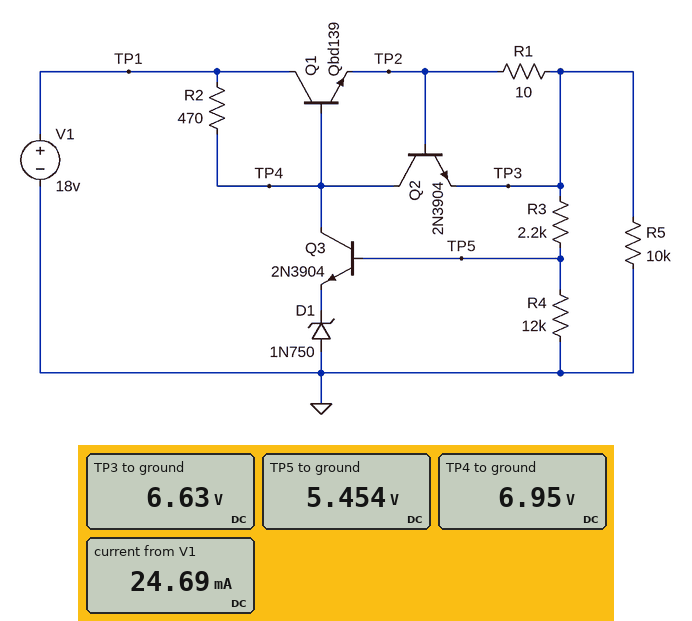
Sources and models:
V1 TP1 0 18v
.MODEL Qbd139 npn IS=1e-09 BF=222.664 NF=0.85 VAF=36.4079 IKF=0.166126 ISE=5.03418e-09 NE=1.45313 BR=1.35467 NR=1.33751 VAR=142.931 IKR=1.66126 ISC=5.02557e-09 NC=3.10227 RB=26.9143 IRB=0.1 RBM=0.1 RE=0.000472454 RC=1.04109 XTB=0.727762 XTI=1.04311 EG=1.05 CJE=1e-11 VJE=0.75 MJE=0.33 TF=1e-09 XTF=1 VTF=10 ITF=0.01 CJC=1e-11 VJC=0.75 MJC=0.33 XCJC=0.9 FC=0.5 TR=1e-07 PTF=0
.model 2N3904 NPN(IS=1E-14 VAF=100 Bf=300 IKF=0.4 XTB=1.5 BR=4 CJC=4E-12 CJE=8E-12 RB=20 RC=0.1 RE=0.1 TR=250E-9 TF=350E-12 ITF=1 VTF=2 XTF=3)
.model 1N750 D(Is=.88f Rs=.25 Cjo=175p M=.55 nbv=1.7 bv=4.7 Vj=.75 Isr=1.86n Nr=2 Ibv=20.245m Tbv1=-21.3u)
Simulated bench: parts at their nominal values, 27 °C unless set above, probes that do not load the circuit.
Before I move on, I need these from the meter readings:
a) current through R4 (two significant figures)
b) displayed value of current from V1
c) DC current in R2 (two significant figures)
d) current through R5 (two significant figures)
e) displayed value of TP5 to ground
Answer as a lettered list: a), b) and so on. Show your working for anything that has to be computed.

a) (5.454 V) / 12 kΩ = 450 µA
b) 24.69 mA
c) (18 V - 6.95 V) / 470 Ω = 24 mA
d) (6.63 V) / 10 kΩ = 660 µA
e) 5.454 V
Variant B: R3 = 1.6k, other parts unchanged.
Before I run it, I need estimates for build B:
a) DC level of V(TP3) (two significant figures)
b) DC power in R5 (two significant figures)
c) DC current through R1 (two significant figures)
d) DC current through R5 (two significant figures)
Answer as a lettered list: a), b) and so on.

a) 6.3 V
b) 4.0 mW
c) 1.2 mA
d) 630 µA
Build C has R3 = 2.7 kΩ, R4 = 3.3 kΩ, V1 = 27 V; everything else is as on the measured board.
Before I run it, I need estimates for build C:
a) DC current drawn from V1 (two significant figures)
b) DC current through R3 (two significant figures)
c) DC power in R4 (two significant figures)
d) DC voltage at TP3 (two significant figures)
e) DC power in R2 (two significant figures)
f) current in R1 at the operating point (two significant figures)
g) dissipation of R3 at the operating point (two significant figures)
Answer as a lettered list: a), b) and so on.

a) 38 mA
b) 1.8 mA
c) 9.1 mW
d) 10 V
e) 570 mW
f) 2.8 mA
g) 8.6 mW
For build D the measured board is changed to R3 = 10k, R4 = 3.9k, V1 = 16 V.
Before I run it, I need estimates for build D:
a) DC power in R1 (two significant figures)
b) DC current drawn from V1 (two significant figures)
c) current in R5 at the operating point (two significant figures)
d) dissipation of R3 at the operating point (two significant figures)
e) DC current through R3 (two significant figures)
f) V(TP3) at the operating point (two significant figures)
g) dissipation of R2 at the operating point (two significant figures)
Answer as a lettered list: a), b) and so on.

a) 72 µW
b) 2.7 mA
c) 1.6 mA
d) 13 mW
e) 1.1 mA
f) 16 V
g) 800 nW
